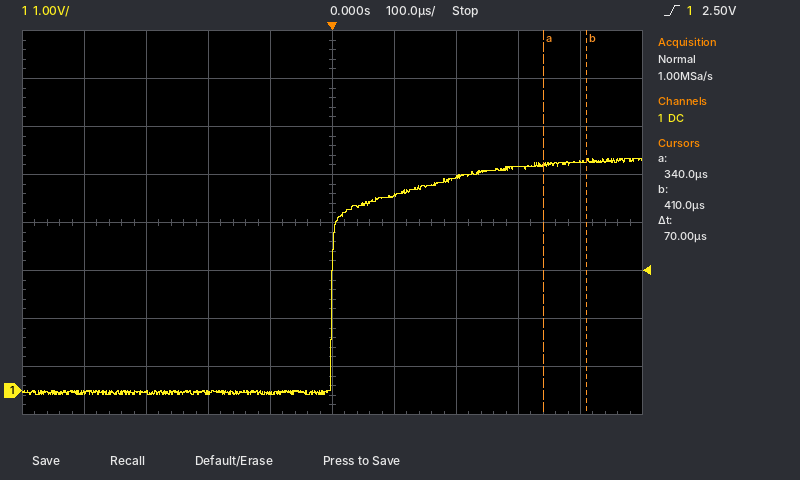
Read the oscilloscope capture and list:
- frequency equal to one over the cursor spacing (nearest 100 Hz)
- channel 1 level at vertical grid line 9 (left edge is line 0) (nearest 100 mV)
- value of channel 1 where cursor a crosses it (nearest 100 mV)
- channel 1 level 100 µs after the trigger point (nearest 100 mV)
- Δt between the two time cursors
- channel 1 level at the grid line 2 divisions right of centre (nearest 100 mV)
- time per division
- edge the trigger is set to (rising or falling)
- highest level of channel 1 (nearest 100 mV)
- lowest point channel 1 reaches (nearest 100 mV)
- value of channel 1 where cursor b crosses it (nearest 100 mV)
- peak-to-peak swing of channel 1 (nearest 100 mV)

14.3 kHz
4.8 V
4.7 V
4.1 V
70 µs
4.5 V
100 µs
rising
4.8 V
-100 mV
4.8 V
4.9 V
